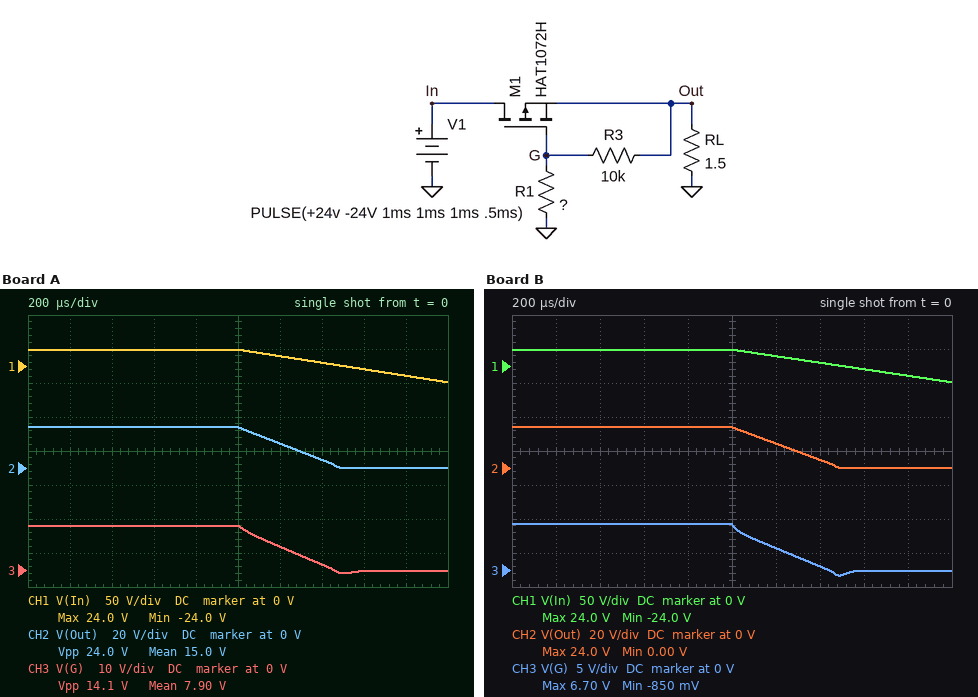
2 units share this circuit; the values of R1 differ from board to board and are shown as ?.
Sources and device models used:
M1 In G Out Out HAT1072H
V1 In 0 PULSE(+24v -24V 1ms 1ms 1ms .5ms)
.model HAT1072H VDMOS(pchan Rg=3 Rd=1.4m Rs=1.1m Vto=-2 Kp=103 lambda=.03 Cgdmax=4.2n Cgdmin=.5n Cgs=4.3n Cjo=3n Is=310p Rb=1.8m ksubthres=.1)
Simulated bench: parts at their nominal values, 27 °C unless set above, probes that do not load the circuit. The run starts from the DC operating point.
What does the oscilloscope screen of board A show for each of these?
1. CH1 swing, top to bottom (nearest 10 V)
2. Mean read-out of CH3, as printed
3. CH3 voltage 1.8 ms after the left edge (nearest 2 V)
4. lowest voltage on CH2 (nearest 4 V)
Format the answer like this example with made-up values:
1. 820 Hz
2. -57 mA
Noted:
1. 50 V
2. 7.90 V
3. 0 V
4. 0 V
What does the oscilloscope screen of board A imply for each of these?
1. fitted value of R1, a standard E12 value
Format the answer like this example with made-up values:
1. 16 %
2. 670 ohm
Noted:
1. 12 kΩ
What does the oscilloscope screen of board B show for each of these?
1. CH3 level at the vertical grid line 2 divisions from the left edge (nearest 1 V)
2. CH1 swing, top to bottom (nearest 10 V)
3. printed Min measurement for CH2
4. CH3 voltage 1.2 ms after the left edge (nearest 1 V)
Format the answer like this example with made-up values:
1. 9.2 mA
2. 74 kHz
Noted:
1. 7 V
2. 50 V
3. 0.00 V
4. 3 V
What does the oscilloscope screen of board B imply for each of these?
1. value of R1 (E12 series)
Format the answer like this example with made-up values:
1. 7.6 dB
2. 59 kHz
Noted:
1. 3.9 kΩ
